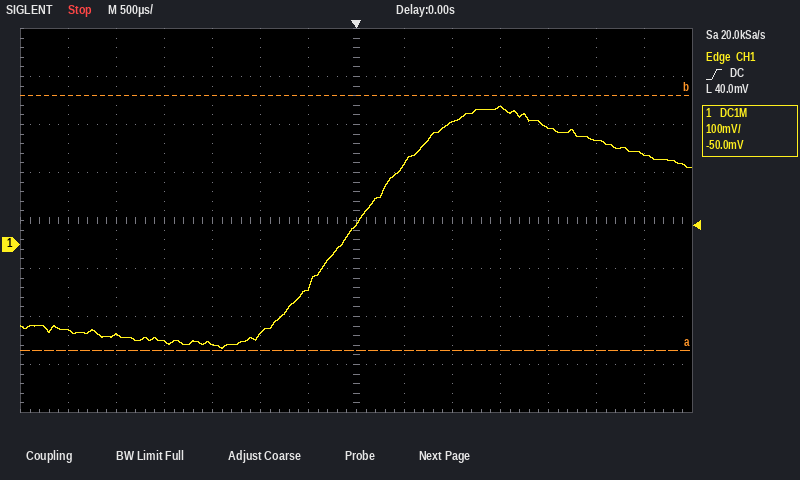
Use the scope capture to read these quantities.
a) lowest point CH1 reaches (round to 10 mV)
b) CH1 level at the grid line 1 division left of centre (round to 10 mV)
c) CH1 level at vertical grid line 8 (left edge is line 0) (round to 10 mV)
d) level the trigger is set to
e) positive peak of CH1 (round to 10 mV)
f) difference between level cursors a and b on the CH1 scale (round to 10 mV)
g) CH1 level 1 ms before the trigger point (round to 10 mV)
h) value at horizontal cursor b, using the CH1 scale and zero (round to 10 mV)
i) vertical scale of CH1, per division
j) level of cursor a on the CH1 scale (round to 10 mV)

-220 mV
-90 mV
170 mV
40.0 mV
290 mV
530 mV
-190 mV
310 mV
100 mV
-220 mV
